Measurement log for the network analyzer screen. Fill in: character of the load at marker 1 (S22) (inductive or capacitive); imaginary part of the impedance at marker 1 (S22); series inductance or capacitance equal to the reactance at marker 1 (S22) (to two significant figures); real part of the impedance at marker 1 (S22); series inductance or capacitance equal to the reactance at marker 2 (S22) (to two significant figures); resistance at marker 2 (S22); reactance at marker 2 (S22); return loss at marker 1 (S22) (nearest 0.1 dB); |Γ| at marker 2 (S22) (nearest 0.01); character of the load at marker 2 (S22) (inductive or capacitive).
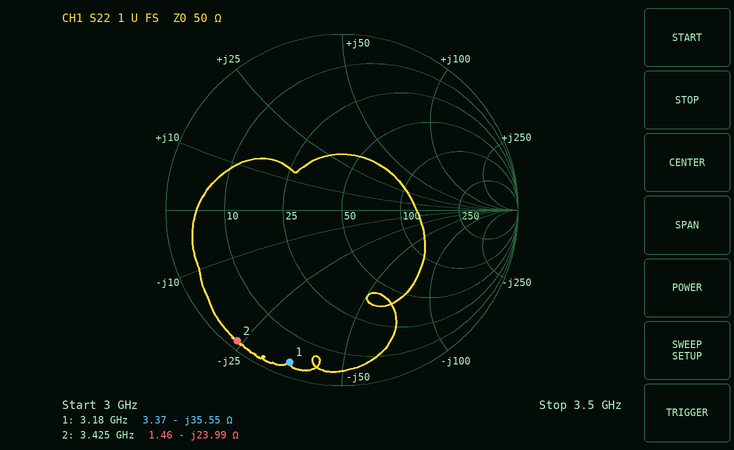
capacitive
-35.55 Ω
1.4 pF
3.37 Ω
1.9 pF
1.46 Ω
-23.99 Ω
0.8 dB
0.95
capacitive
